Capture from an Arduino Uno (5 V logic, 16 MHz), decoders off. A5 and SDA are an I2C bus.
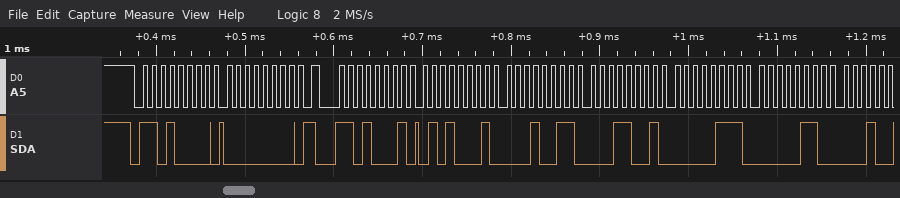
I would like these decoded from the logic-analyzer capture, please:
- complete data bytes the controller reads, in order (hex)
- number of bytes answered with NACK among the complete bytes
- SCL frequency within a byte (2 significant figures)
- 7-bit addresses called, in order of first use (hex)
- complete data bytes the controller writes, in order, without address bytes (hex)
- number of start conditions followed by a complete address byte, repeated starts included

51 13 19 07 06
0
100 kHz
0x68
00
2
